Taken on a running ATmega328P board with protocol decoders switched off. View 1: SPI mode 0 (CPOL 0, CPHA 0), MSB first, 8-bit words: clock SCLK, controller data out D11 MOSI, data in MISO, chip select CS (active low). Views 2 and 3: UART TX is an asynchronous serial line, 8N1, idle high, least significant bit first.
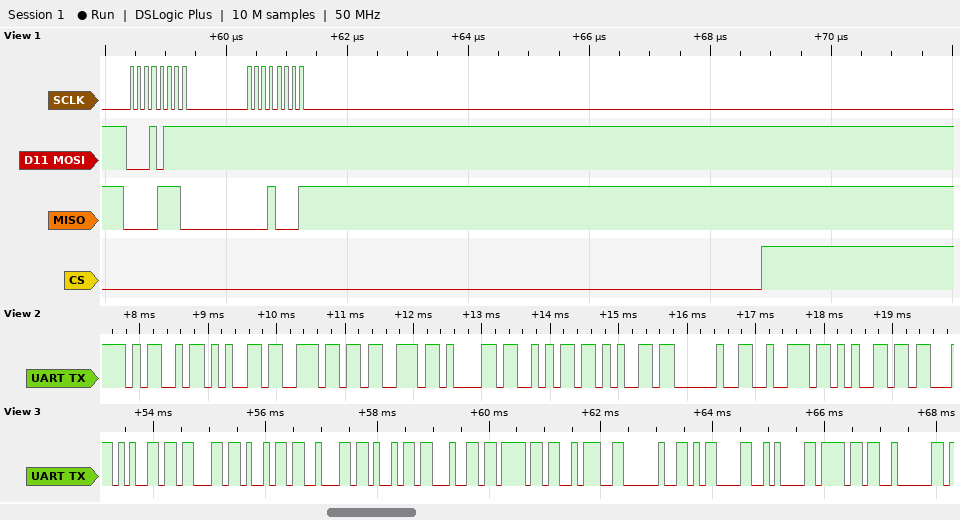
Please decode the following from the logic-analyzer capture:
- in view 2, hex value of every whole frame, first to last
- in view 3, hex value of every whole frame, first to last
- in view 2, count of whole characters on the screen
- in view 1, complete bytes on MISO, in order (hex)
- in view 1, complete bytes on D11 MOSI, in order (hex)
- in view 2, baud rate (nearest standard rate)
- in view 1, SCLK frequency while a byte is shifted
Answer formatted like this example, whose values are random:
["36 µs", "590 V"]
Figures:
["4D 65 6E 73 61 6A 65 20 72 65", "0x65 0x63 0x69 0x62 0x69 0x64 0x6F 0x3A 0x20 0x0D 0x0A 0x6F 0x02", "10", "0x0E 0x11", "0x17 0xFF", "9600 baud", "8 MHz"]
